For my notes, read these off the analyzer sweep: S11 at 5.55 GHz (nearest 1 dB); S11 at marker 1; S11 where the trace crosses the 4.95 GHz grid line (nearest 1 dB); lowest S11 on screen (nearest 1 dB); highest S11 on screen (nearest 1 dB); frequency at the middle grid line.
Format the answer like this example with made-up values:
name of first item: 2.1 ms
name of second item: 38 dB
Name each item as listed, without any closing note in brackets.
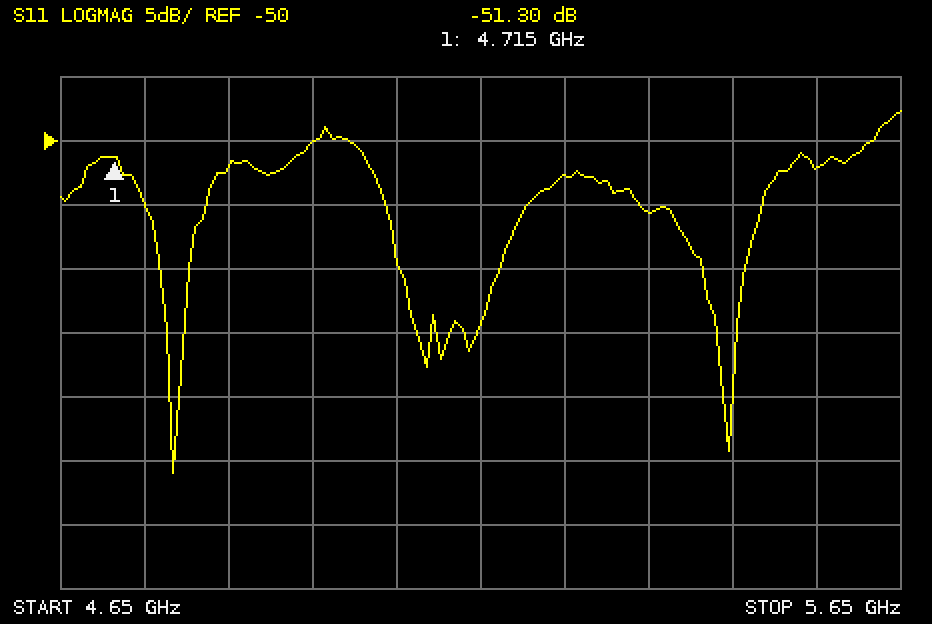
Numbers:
S11 at 5.55 GHz: -52 dB
S11 at marker 1: -51.30 dB
S11 where the trace crosses the 4.95 GHz grid line: -50 dB
lowest S11 on screen: -76 dB
highest S11 on screen: -48 dB
frequency at the middle grid line: 5.15 GHz
